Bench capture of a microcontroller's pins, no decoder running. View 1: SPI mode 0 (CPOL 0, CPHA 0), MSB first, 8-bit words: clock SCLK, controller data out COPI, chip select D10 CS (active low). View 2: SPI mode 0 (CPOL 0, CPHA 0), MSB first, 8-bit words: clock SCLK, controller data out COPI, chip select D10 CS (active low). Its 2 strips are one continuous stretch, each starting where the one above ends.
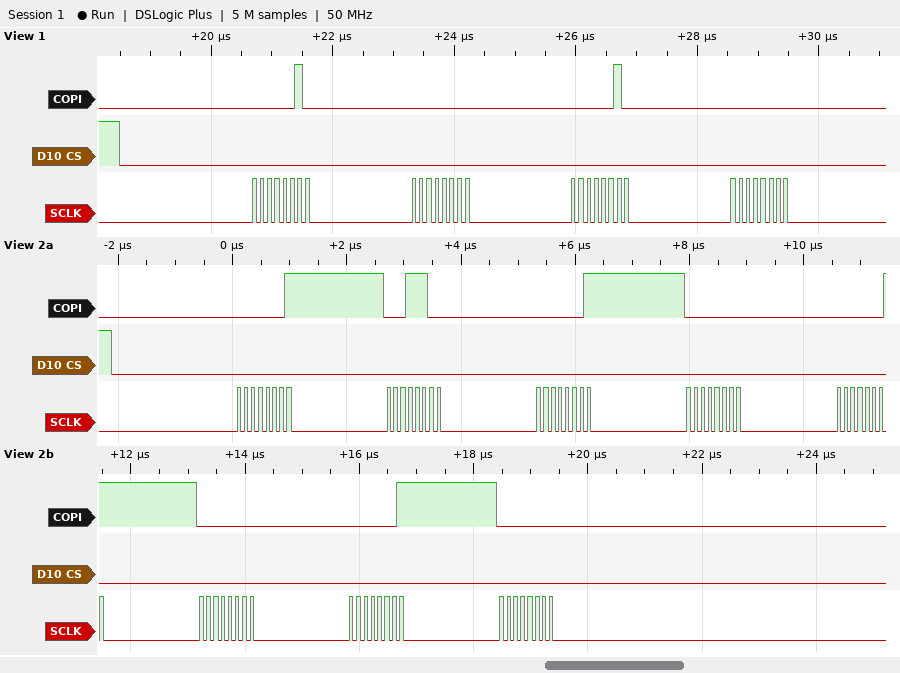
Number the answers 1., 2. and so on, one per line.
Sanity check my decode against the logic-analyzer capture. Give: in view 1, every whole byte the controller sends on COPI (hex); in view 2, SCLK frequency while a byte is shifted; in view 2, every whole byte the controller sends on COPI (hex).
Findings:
1. 02 00 02 00
2. 8 MHz
3. 0x01 0x1C 0x01 0x00 0x01 0x00 0x01 0x00
